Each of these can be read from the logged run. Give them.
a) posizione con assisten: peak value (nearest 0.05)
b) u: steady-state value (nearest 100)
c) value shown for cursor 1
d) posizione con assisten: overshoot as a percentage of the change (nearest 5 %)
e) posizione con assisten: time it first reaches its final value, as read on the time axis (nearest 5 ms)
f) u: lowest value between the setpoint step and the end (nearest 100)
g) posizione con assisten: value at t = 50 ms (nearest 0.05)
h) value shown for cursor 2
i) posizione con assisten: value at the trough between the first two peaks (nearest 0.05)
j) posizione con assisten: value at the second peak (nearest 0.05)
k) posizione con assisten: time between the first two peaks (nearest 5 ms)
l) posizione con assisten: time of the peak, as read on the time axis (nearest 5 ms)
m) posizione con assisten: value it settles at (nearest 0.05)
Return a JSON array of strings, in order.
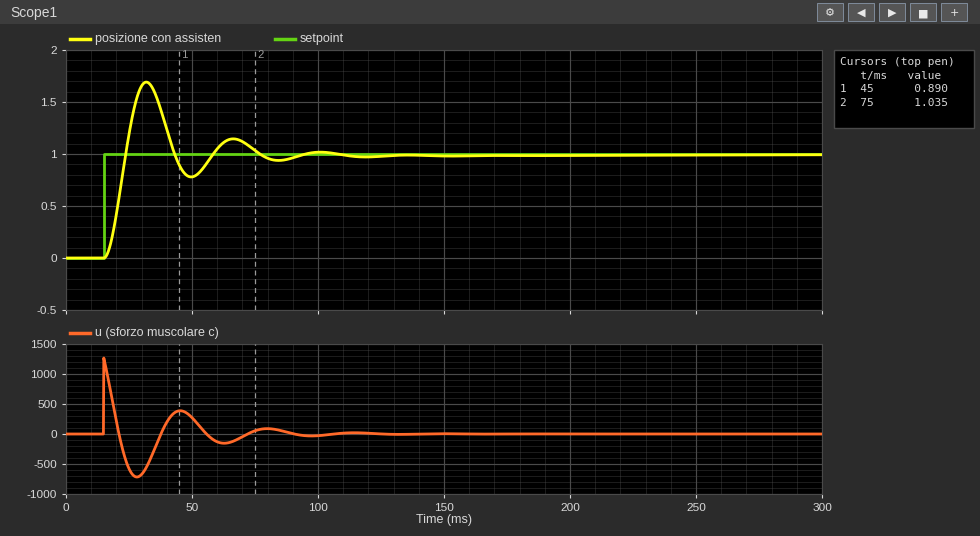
["1.70", "0", "0.890", "70 %", "25 ms", "-700", "0.80", "1.035", "0.80", "1.15", "35 ms", "30 ms", "1.00"]
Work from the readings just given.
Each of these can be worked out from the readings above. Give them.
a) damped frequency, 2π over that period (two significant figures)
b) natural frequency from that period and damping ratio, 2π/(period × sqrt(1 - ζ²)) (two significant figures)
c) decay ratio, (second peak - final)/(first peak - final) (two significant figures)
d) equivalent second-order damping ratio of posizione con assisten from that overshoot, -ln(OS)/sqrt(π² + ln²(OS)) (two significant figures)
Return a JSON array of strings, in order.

["0.18 rad/ms", "0.18 rad/ms", "0.21", "0.11"]
